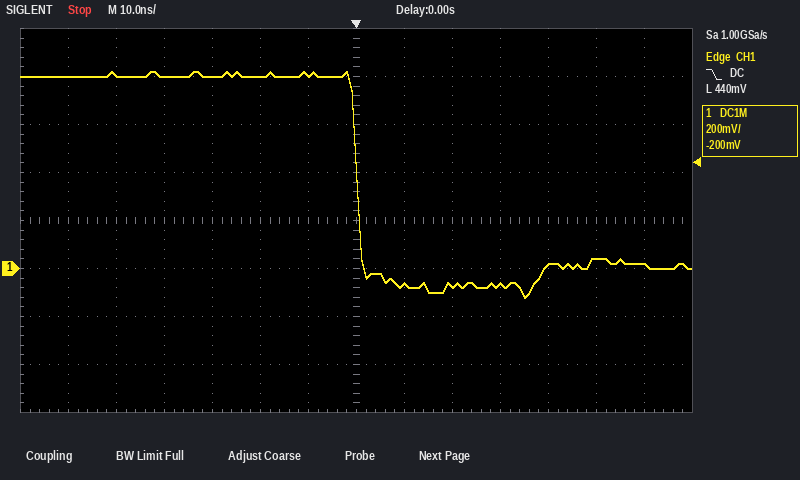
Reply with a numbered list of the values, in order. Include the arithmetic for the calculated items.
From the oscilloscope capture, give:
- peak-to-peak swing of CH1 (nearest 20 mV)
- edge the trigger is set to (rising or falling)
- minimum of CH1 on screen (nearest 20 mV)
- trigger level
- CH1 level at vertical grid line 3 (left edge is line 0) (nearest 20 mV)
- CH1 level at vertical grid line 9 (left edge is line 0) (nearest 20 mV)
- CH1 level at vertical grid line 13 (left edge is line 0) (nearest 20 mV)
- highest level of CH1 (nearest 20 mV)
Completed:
1. 820 mV − (-120 mV) = 940 mV
2. falling
3. -120 mV
4. 440 mV
5. 800 mV
6. -80 mV
7. 20 mV
8. 820 mV
